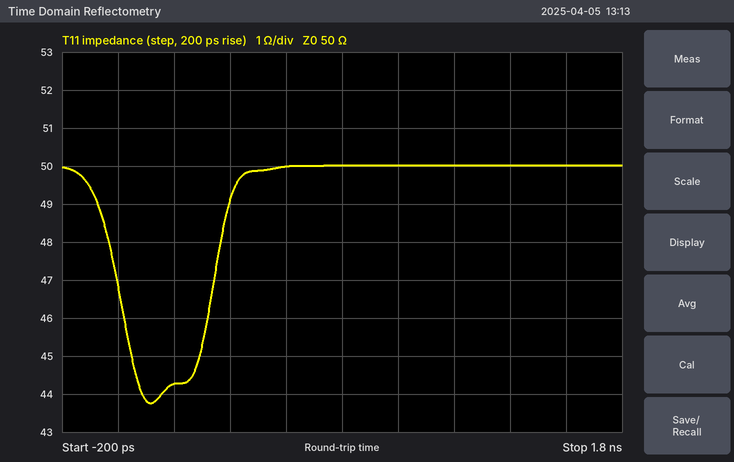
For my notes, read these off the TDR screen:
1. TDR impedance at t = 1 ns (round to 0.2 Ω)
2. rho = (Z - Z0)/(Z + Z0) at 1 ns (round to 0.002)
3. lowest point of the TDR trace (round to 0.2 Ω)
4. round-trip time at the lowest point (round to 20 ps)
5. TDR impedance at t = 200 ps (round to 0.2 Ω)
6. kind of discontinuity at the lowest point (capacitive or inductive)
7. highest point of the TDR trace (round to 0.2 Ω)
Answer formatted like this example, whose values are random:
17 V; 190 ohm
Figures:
50.0 Ω; 0.000; 43.8 Ω; 120 ps; 44.2 Ω; capacitive; 50.0 Ω
